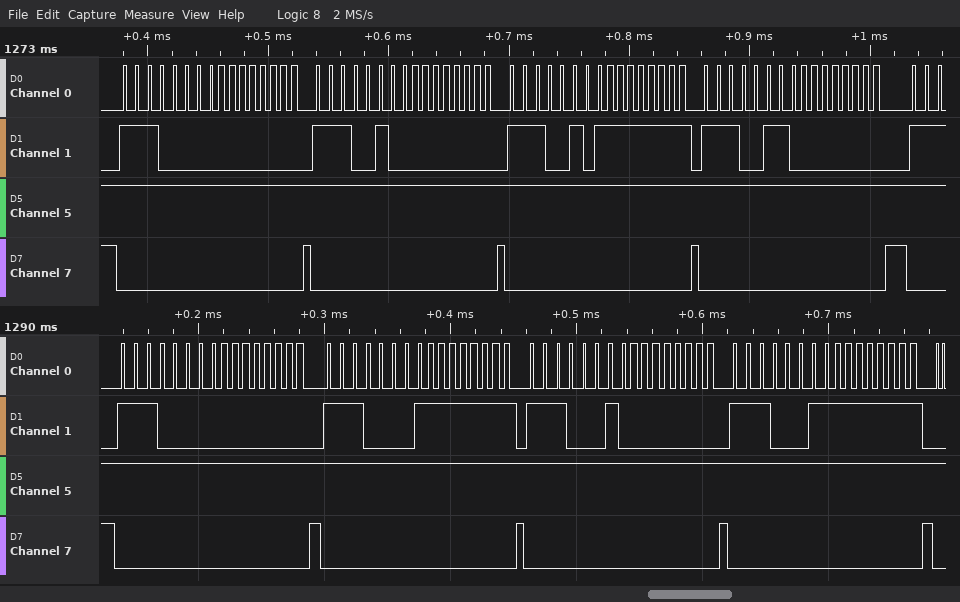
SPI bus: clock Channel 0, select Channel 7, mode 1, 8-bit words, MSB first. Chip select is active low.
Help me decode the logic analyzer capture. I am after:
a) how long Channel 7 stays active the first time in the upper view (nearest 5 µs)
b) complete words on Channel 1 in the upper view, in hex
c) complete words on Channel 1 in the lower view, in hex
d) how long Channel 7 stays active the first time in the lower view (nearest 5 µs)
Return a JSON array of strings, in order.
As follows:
["155 µs", "E0, 00, E4, 00, E5, FF, E6, 00", "E0, 00, E1, FF, E2, 00, E3, FF", "155 µs"]
